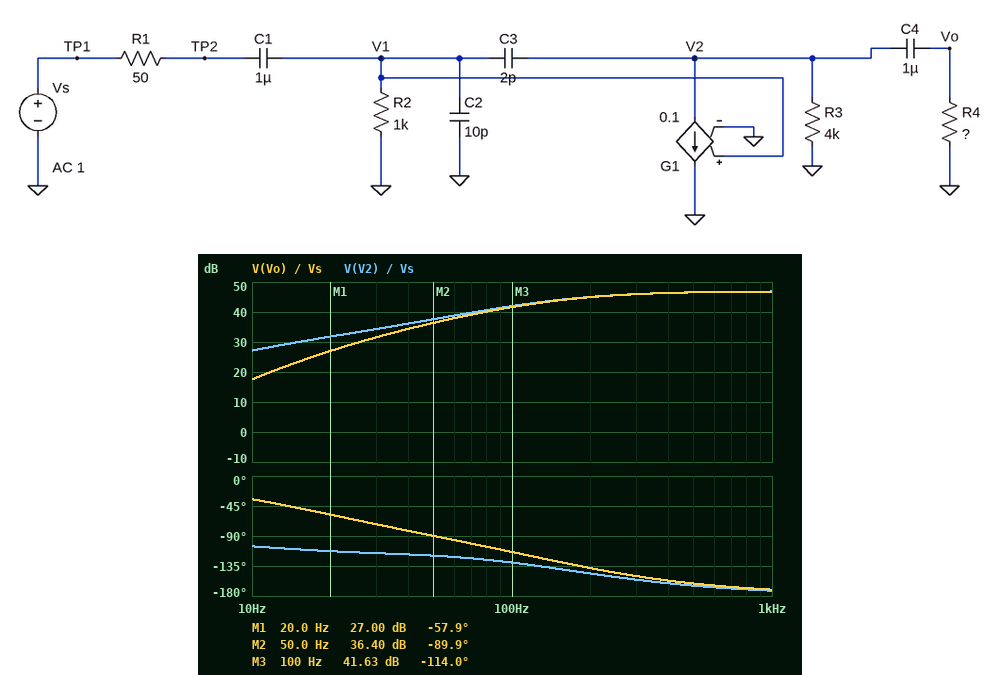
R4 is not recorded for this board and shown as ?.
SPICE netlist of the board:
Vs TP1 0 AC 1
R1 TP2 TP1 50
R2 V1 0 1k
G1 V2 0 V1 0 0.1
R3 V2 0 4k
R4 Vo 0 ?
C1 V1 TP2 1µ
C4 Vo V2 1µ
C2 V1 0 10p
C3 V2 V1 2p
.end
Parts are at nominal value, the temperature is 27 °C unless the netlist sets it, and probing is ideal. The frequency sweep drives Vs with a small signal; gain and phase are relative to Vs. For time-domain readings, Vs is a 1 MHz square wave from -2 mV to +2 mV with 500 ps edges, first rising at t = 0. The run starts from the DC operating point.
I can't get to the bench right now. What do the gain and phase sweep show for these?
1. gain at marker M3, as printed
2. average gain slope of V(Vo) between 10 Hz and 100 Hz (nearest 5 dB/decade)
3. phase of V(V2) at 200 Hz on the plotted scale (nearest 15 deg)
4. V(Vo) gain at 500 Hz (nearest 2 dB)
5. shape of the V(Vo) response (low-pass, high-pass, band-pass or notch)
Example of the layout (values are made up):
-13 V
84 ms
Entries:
41.63 dB
25 dB/decade
-150 deg
46 dB
high-pass
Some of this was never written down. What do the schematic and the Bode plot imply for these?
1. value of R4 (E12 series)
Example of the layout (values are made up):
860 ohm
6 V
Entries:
5.6 kΩ
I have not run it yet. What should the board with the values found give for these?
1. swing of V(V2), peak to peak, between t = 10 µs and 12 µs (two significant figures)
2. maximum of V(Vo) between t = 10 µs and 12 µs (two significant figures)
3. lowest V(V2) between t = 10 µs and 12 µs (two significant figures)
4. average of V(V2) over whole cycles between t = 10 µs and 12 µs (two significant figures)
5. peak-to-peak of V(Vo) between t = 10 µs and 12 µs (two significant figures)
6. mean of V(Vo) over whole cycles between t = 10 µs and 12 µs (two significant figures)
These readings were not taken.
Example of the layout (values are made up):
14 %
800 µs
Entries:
890 mV
5.6 mV
-880 mV
-440 mV
890 mV
-440 mV
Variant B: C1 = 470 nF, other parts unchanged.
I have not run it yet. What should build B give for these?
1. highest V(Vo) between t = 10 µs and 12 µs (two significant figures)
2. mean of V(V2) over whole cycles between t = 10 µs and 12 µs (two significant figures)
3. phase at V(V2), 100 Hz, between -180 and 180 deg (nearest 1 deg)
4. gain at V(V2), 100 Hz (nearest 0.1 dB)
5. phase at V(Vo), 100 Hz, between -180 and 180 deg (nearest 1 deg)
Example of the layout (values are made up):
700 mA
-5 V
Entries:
11 mV
-430 mV
-114 deg
36.6 dB
-98 deg
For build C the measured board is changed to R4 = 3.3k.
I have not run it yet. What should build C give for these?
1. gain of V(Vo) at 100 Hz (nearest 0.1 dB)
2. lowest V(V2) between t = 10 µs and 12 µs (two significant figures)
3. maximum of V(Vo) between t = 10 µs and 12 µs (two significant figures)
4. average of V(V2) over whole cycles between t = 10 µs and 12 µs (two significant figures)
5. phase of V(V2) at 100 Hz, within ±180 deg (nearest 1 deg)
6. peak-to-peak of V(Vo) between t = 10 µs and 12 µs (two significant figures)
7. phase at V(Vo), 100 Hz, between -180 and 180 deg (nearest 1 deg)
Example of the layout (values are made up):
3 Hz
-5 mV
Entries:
39.3 dB
-690 mV
4.5 mV
-340 mV
-137 deg
690 mV
-111 deg
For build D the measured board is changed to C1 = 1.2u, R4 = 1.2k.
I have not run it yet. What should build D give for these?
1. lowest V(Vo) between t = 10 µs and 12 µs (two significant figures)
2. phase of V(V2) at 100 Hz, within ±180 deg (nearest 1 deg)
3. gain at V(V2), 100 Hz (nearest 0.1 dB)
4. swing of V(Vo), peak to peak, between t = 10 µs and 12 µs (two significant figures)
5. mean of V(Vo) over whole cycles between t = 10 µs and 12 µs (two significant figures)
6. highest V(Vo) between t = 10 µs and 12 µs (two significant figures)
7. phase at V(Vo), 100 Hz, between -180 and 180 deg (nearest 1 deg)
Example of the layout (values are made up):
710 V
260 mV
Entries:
-350 mV
-164 deg
38.8 dB
350 mV
-170 mV
2.1 mV
-111 deg
